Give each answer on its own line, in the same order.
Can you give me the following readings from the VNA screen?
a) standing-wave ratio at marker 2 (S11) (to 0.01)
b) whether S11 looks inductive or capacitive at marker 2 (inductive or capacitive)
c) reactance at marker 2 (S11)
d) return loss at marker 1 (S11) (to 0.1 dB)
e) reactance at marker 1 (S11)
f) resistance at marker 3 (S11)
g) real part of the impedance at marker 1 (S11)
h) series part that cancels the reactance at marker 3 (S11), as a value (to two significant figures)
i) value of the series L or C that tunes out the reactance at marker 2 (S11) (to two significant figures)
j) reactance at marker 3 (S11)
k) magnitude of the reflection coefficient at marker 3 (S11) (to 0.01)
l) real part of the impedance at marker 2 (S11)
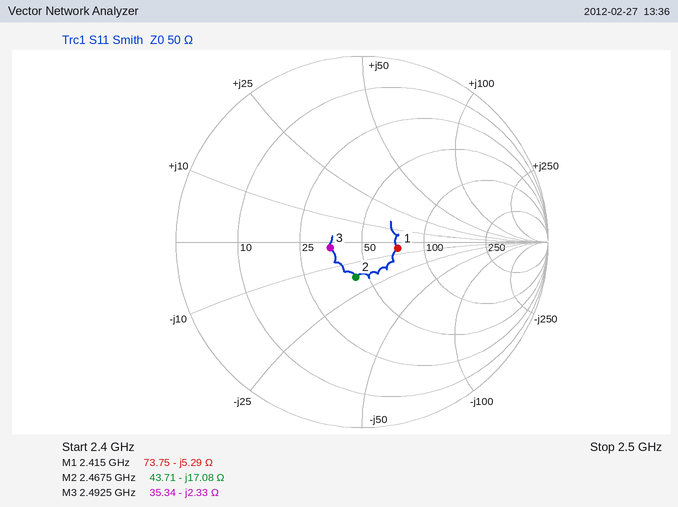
1.47
capacitive
-17.08 Ω
14.1 dB
-5.29 Ω
35.34 Ω
73.75 Ω
150 pH
1.1 nH
-2.33 Ω
0.17
43.71 Ω
